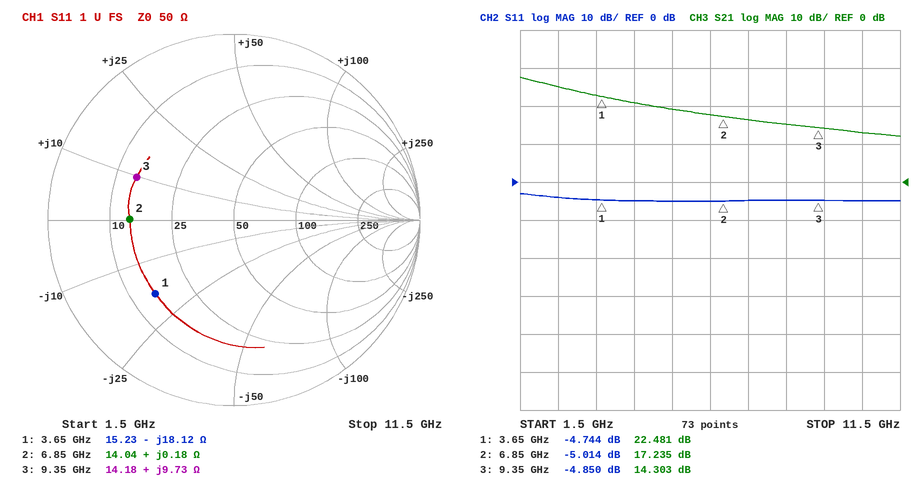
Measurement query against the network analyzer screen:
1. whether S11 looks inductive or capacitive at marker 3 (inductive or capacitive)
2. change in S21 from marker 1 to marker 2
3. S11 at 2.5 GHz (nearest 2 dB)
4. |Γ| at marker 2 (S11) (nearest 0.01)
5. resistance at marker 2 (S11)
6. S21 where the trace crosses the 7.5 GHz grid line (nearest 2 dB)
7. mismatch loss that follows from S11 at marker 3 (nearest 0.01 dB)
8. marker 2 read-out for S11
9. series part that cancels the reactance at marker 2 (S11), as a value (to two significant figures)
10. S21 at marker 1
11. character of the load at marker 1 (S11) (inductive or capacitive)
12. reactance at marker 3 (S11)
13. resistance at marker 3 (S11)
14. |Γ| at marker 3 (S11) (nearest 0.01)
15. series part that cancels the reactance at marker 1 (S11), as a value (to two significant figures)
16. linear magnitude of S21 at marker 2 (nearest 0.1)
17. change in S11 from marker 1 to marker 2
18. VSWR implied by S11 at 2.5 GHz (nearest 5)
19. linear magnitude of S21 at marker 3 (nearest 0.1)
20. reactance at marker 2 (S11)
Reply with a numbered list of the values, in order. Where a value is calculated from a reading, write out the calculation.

1. inductive
2. 17.235 − (22.481) = -5.246 dB
3. -4 dB
4. 0.56
5. 14.04 Ω
6. 16 dB
7. −10 log10(1 − 10^(-4.85/10)) ≈ 1.72 dB
8. -5.014 dB
9. C = 1/(2π × 6.85 GHz × 0.18 Ω) ≈ 129 pF, so 130 pF to two significant figures
10. 22.481 dB
11. capacitive
12. +9.73 Ω
13. 14.18 Ω
14. 0.57
15. L = 18.12 Ω/(2π × 3.65 GHz) ≈ 790 pH
16. 10^(17.235/20) ≈ 7.3
17. -5.014 − (-4.744) = -0.270 dB
18. |Γ| = 10^(-4/20) = 0.6310; VSWR = (1 + 0.6310)/(1 − 0.6310) ≈ 4.42, so 5 to the nearest 5
19. 10^(14.303/20) ≈ 5.2
20. +0.18 Ω
